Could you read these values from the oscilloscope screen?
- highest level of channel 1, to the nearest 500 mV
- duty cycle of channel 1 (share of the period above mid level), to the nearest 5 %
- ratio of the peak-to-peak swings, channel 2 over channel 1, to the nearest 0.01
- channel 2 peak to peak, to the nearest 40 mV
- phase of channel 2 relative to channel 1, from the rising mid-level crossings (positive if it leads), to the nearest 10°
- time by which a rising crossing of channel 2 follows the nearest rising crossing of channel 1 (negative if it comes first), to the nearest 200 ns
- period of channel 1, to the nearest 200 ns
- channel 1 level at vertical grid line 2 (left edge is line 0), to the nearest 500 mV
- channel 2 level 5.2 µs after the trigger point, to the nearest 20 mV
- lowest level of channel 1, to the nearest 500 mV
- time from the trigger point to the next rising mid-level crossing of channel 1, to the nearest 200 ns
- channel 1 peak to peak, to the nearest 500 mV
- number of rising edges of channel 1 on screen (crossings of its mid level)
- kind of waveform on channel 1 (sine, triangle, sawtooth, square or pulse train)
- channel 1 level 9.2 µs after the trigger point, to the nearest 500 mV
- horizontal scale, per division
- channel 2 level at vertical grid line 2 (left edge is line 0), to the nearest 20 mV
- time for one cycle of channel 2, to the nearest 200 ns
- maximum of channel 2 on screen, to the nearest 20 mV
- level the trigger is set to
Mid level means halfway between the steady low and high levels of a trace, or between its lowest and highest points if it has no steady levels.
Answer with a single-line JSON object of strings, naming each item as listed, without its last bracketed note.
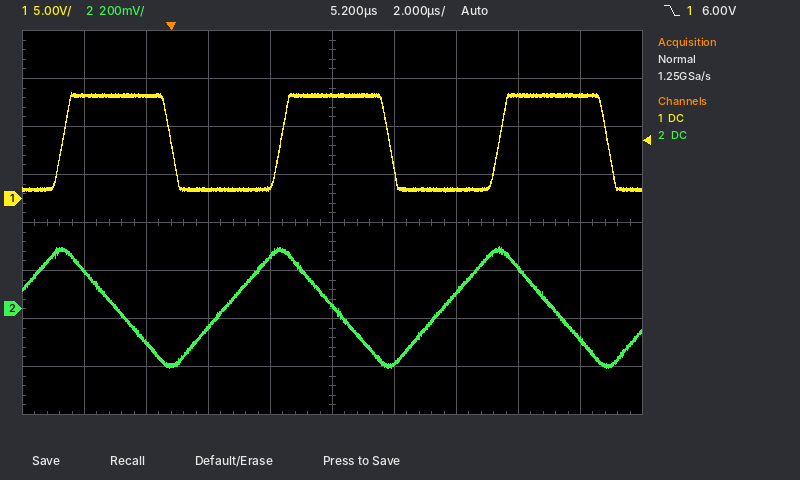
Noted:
{"highest level of channel 1, to the nearest 500 mV": "11.0 V", "duty cycle of channel 1 (share of the period above mid level), to the nearest 5 %": "50 %", "ratio of the peak-to-peak swings, channel 2 over channel 1, to the nearest 0.01": "0.05", "channel 2 peak to peak, to the nearest 40 mV": "520 mV", "phase of channel 2 relative to channel 1, from the rising mid-level crossings (positive if it leads), to the nearest 10°": "+90°", "time by which a rising crossing of channel 2 follows the nearest rising crossing of channel 1 (negative if it comes first), to the nearest 200 ns": "-1.8 µs", "period of channel 1, to the nearest 200 ns": "7.0 µs", "channel 1 level at vertical grid line 2 (left edge is line 0), to the nearest 500 mV": "10.5 V", "channel 2 level 5.2 µs after the trigger point, to the nearest 20 mV": "20 mV", "lowest level of channel 1, to the nearest 500 mV": "500 mV", "time from the trigger point to the next rising mid-level crossing of channel 1, to the nearest 200 ns": "3.6 µs", "channel 1 peak to peak, to the nearest 500 mV": "10.5 V", "number of rising edges of channel 1 on screen": "3", "kind of waveform on channel 1": "square", "channel 1 level 9.2 µs after the trigger point, to the nearest 500 mV": "1.0 V", "horizontal scale, per division": "2 µs", "channel 2 level at vertical grid line 2 (left edge is line 0), to the nearest 20 mV": "-140 mV", "time for one cycle of channel 2, to the nearest 200 ns": "7.0 µs", "maximum of channel 2 on screen, to the nearest 20 mV": "260 mV", "level the trigger is set to": "6.00 V"}
